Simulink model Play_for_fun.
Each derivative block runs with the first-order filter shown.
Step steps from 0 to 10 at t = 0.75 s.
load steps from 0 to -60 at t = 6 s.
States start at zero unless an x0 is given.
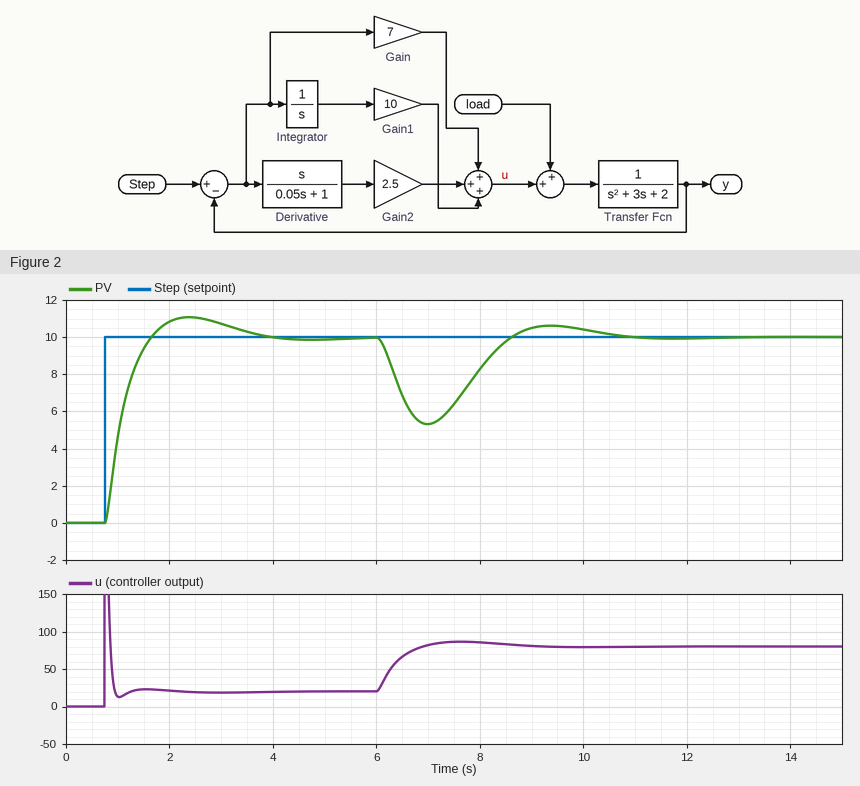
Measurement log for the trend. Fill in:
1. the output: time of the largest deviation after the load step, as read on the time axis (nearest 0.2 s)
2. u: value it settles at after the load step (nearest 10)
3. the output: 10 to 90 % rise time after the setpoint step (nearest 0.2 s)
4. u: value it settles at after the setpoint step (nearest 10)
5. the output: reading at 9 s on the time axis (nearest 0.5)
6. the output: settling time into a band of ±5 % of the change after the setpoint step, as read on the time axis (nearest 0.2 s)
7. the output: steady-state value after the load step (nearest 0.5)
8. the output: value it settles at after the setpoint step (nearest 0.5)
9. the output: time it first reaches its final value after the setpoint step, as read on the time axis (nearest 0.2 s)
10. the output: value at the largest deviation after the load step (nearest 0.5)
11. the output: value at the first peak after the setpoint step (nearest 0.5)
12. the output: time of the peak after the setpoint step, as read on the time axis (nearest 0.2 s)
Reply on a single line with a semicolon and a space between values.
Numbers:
7.0 s; 80; 0.6 s; 20; 10.5; 3.2 s; 10.0; 10.0; 1.6 s; 5.5; 11.0; 2.4 s
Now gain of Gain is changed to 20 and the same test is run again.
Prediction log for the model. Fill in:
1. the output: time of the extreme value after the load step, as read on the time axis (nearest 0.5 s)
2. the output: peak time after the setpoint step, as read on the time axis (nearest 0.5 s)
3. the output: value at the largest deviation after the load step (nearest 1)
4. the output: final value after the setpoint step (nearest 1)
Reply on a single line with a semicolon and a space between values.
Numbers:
6.5 s; 1.5 s; 7; 10
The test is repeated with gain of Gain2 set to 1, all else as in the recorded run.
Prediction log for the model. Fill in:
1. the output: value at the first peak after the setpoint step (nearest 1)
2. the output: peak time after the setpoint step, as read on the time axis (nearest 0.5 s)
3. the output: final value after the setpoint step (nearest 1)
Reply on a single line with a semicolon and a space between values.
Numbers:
12; 2.0 s; 10
